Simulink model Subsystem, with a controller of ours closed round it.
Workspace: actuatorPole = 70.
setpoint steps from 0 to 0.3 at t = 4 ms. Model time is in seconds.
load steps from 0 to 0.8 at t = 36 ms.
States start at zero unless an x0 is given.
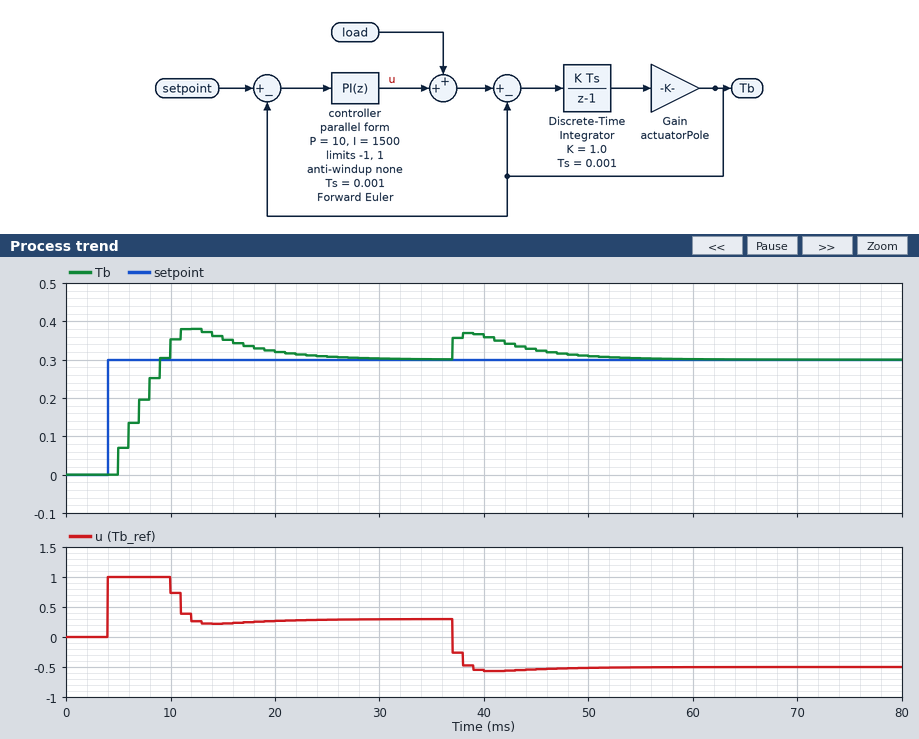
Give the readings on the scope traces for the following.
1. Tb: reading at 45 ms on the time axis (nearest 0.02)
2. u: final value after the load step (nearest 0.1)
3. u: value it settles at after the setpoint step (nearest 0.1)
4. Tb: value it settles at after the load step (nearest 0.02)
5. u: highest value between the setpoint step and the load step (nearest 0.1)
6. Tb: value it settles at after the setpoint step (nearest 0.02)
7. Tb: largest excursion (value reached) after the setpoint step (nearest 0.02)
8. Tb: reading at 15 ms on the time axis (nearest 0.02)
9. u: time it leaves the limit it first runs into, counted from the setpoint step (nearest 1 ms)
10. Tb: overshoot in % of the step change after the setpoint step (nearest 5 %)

0.32
-0.5
0.3
0.30
1.0
0.30
0.38
0.36
6 ms
25 %
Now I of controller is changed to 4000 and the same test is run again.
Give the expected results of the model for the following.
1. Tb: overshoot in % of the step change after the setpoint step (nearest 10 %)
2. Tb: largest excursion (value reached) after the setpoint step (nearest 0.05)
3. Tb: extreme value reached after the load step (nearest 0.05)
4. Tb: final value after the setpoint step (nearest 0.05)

60 %
0.50
0.35
0.30
